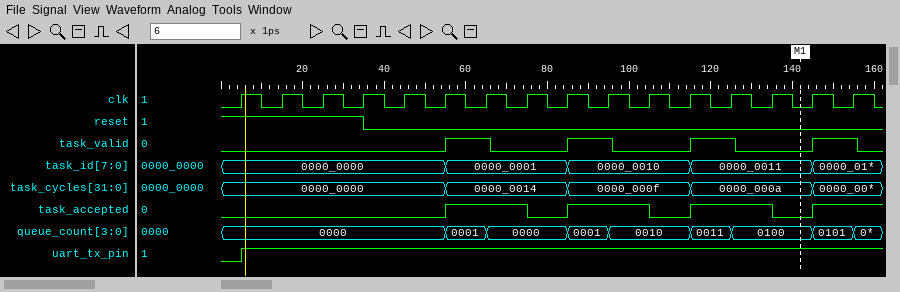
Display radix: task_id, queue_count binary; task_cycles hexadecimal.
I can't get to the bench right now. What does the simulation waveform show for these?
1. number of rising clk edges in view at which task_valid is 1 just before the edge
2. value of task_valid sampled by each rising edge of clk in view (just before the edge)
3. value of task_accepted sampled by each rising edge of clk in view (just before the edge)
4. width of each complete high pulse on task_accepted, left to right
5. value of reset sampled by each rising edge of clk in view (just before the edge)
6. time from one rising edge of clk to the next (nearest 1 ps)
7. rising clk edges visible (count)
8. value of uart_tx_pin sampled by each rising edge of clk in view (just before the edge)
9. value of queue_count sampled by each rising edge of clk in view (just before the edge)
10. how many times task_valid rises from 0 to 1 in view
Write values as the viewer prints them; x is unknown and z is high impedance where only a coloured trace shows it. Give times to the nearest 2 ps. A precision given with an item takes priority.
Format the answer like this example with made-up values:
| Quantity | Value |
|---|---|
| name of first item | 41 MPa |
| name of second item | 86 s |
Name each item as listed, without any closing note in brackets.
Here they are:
| Quantity | Value |
|---|---|
| number of rising clk edges in view at which task_valid is 1 just before the edge | 4 |
| value of task_valid sampled by each rising edge of clk in view | 0 0 0 0 0 0 1 0 0 1 0 0 1 0 0 1 |
| value of task_accepted sampled by each rising edge of clk in view | 0 0 0 0 0 0 1 1 0 1 1 0 1 1 0 1 |
| width of each complete high pulse on task_accepted, left to right | 20 ps, 20 ps, 20 ps |
| value of reset sampled by each rising edge of clk in view | 1 1 1 1 0 0 0 0 0 0 0 0 0 0 0 0 |
| time from one rising edge of clk to the next | 10 ps |
| rising clk edges visible | 16 |
| value of uart_tx_pin sampled by each rising edge of clk in view | 0 1 1 1 1 1 1 1 1 1 1 1 1 1 1 1 |
| value of queue_count sampled by each rising edge of clk in view | 0000, 0000, 0000, 0000, 0000, 0000, 0001, 0000, 0000, 0001, 0010, 0010, 0011, 0100, 0100, 0101 |
| how many times task_valid rises from 0 to 1 in view | 4 |
